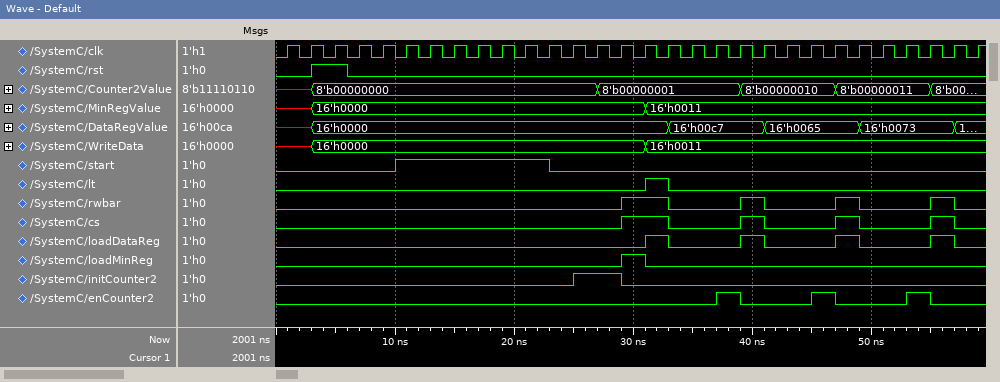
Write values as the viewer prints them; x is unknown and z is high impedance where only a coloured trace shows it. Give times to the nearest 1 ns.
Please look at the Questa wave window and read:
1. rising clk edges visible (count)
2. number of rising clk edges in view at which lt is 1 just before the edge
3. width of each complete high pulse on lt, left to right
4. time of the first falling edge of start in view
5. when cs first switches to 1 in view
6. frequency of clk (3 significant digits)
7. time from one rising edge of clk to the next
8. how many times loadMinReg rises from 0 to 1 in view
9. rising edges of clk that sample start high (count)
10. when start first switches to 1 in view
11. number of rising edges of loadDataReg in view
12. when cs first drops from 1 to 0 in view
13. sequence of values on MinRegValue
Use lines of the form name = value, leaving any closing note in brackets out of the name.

rising clk edges visible = 30
number of rising clk edges in view at which lt is 1 just before the edge = 1
width of each complete high pulse on lt, left to right = 2 ns
time of the first falling edge of start in view = 23 ns
when cs first switches to 1 in view = 29 ns
frequency of clk = 500 MHz
time from one rising edge of clk to the next = 2 ns
how many times loadMinReg rises from 0 to 1 in view = 1
rising edges of clk that sample start high = 7
when start first switches to 1 in view = 10 ns
number of rising edges of loadDataReg in view = 4
when cs first drops from 1 to 0 in view = 33 ns
sequence of values on MinRegValue = x, 16'h0000, 16'h0011
